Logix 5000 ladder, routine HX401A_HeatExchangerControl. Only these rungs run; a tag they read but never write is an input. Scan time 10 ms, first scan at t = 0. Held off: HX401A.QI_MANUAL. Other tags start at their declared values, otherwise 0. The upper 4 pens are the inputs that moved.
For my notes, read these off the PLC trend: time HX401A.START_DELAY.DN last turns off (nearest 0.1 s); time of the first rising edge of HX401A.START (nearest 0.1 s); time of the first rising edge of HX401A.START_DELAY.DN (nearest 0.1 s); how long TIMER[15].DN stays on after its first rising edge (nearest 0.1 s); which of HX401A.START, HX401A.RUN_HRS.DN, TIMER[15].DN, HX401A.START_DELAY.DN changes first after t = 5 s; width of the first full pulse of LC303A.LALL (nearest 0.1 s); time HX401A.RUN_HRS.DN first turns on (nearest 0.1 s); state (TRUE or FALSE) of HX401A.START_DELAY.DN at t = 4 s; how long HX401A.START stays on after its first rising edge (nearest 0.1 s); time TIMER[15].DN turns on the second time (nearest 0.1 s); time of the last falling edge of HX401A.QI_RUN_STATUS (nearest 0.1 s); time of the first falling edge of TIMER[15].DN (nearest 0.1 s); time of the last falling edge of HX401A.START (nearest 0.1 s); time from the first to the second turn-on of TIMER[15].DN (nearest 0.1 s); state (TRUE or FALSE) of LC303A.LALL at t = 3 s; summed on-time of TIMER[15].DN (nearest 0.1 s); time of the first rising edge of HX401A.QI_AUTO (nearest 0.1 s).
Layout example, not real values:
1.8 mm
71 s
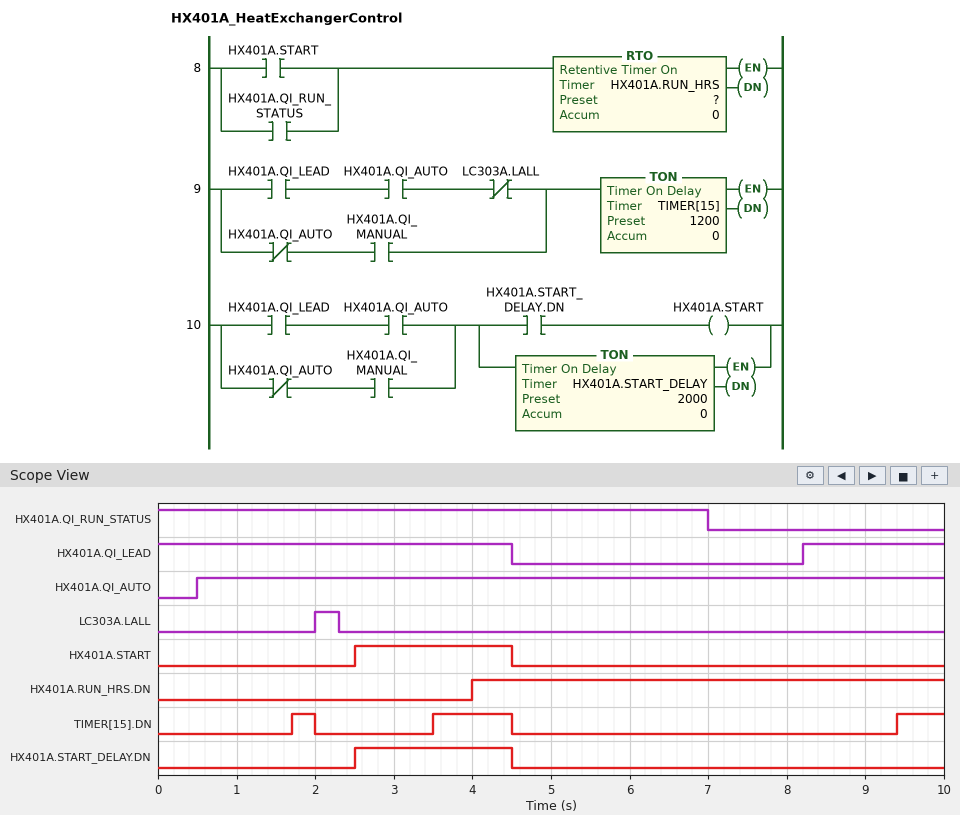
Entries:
4.5 s
2.5 s
2.5 s
0.3 s
TIMER[15].DN
0.3 s
4.0 s
TRUE
2.0 s
3.5 s
7.0 s
2.0 s
4.5 s
1.8 s
FALSE
1.9 s
0.5 s
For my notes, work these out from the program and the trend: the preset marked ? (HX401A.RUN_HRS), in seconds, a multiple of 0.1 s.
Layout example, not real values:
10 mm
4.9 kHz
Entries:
4.0 s
